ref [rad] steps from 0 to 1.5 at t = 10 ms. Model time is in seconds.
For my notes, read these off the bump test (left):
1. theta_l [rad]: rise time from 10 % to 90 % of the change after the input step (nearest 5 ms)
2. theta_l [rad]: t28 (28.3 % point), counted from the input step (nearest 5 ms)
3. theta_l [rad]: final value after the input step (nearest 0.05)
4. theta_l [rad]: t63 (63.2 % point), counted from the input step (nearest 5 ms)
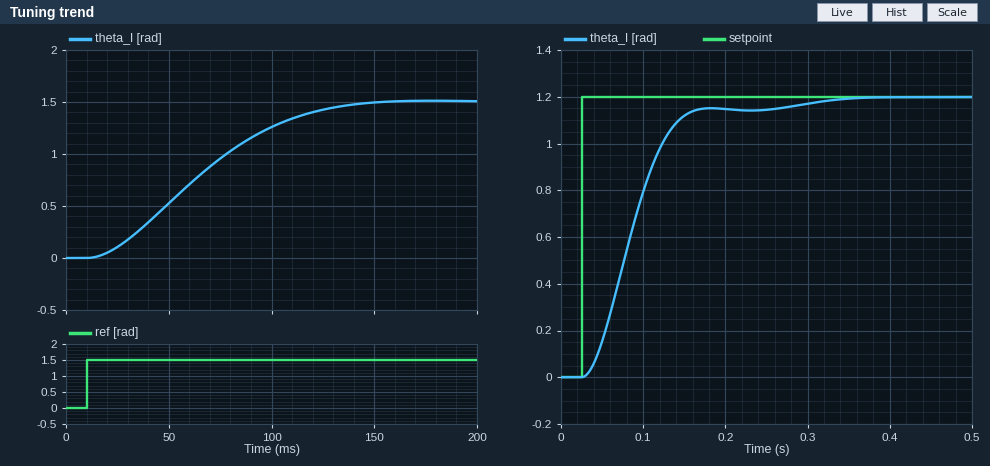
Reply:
85 ms
35 ms
1.50
65 ms
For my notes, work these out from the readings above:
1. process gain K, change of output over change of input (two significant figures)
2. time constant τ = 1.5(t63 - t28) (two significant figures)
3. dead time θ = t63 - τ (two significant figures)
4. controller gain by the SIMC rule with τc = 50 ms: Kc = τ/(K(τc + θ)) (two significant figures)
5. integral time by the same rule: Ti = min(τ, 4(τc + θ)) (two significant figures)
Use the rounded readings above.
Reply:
1.0
45 ms
20 ms
0.64
45 ms
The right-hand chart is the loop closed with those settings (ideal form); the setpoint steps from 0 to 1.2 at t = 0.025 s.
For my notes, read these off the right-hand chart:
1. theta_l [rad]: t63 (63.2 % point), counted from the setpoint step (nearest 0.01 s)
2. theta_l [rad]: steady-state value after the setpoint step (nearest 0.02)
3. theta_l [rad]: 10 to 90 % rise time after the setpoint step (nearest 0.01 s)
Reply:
0.07 s
1.20
0.09 s
